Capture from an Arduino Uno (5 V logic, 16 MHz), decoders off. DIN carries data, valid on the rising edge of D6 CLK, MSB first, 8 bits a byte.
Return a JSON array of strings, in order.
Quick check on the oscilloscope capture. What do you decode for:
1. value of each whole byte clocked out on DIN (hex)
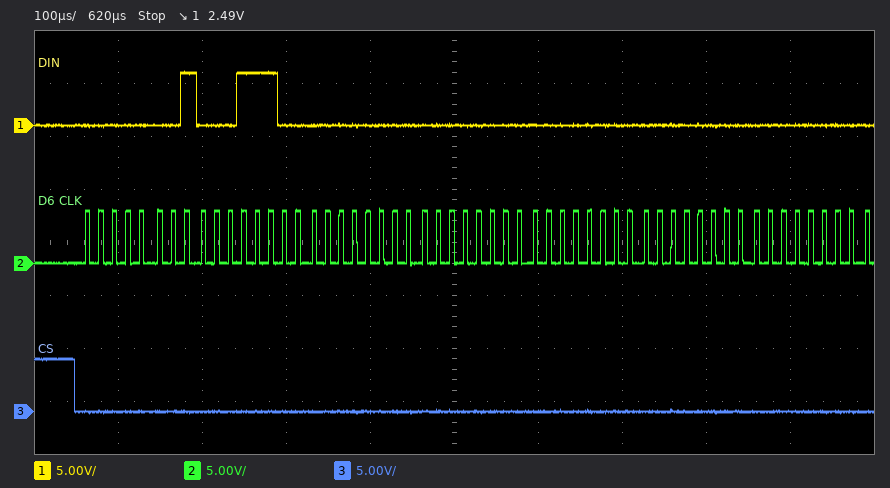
["01 1C 00 00 00 00 00"]
